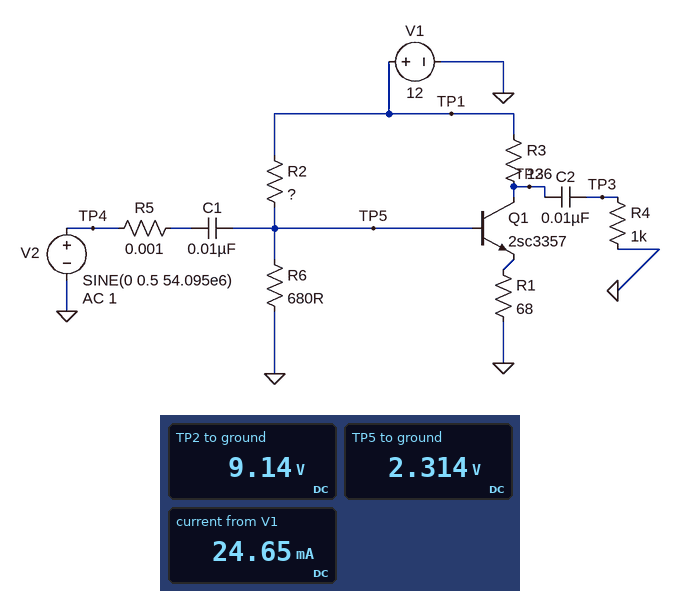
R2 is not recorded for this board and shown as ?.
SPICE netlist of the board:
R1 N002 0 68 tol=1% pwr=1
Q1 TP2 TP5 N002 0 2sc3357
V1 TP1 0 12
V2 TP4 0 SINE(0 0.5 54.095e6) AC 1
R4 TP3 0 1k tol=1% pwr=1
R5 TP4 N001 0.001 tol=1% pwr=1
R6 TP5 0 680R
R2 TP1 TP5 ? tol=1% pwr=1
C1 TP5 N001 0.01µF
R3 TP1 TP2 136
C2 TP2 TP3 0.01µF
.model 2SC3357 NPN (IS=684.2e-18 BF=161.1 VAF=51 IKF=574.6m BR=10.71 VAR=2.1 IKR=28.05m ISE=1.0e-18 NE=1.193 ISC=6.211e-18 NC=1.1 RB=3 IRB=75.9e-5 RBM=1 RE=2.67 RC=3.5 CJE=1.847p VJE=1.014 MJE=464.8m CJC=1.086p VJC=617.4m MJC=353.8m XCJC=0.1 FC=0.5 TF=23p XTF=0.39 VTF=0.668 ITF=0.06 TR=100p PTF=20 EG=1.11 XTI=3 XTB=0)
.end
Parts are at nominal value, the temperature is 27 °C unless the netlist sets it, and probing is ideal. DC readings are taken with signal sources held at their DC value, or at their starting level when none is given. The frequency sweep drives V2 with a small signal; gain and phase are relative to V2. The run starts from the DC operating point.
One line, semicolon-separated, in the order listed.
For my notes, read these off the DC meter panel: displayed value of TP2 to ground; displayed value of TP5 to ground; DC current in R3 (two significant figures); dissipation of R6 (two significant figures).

9.14 V; 2.314 V; 21 mA; 7.9 mW
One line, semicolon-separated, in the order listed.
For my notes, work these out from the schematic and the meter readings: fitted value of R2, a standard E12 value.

2.7 kΩ
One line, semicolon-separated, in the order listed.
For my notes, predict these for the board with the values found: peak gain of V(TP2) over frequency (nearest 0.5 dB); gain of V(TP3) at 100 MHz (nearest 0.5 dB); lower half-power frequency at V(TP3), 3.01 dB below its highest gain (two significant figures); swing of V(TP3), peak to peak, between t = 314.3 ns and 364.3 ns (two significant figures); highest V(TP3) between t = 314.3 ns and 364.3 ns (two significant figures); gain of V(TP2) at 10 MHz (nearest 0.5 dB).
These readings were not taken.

4.5 dB; 4.5 dB; 37 kHz; 1.6 V; 820 mV; 4.5 dB
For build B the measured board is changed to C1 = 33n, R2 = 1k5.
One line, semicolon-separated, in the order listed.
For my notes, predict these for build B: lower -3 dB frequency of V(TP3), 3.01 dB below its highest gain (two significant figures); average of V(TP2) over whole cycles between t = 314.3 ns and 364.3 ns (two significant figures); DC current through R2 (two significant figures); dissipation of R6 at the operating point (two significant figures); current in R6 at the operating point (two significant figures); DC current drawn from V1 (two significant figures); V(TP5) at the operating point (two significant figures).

20 kHz; 6.8 V; 5.6 mA; 19 mW; 5.2 mA; 44 mA; 3.6 V
